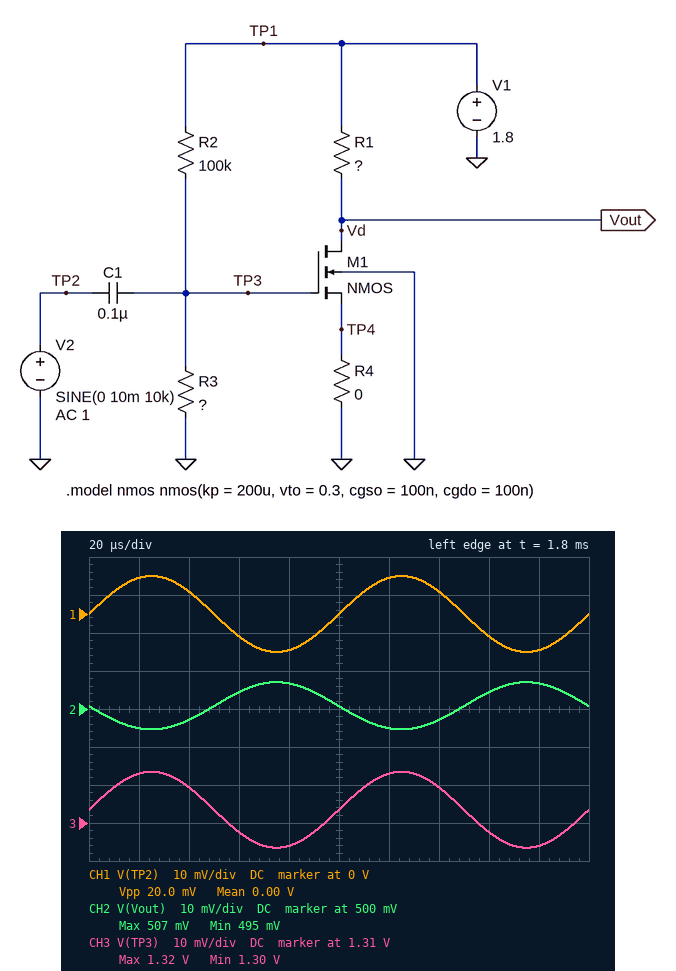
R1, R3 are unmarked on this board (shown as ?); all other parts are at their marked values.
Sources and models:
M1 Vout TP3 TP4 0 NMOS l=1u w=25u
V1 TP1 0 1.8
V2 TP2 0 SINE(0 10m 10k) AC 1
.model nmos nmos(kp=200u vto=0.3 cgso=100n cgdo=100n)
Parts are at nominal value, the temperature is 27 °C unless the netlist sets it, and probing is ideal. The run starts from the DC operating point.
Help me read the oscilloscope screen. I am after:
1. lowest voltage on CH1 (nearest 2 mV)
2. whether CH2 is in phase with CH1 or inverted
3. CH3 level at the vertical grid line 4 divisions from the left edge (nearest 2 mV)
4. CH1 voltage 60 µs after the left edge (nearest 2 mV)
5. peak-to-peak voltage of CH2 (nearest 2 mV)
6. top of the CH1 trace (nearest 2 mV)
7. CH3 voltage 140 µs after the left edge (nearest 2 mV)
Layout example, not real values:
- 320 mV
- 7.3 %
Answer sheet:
- -10 mV
- inverted
- 1.304 V
- -6 mV
- 12 mV
- 10 mV
- 1.320 V
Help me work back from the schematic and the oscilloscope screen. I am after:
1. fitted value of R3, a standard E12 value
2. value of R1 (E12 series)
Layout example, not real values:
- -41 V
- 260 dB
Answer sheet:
- 270 kΩ
- 680 Ω
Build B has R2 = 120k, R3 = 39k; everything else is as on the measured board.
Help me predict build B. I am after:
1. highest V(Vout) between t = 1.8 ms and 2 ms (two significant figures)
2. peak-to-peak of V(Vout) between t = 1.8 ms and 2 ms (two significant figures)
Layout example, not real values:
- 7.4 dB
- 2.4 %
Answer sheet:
- 1.8 V
- 9.6 mV
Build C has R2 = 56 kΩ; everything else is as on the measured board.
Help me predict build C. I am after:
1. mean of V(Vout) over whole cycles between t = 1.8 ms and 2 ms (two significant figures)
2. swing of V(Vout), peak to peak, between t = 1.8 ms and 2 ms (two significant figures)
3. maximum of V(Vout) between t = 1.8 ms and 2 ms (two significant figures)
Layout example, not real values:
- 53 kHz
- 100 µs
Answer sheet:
- 410 mV
- 7.7 mV
- 420 mV
